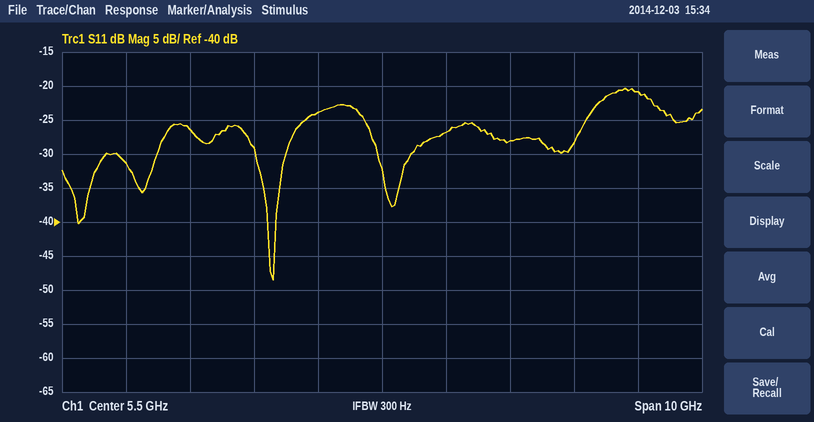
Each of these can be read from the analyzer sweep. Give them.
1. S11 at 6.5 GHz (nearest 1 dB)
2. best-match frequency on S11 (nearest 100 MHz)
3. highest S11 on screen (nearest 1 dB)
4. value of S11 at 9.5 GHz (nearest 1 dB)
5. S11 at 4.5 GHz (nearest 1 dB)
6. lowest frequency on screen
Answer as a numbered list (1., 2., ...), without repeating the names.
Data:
1. -27 dB
2. 3.8 GHz
3. -20 dB
4. -21 dB
5. -24 dB
6. 500 MHz
